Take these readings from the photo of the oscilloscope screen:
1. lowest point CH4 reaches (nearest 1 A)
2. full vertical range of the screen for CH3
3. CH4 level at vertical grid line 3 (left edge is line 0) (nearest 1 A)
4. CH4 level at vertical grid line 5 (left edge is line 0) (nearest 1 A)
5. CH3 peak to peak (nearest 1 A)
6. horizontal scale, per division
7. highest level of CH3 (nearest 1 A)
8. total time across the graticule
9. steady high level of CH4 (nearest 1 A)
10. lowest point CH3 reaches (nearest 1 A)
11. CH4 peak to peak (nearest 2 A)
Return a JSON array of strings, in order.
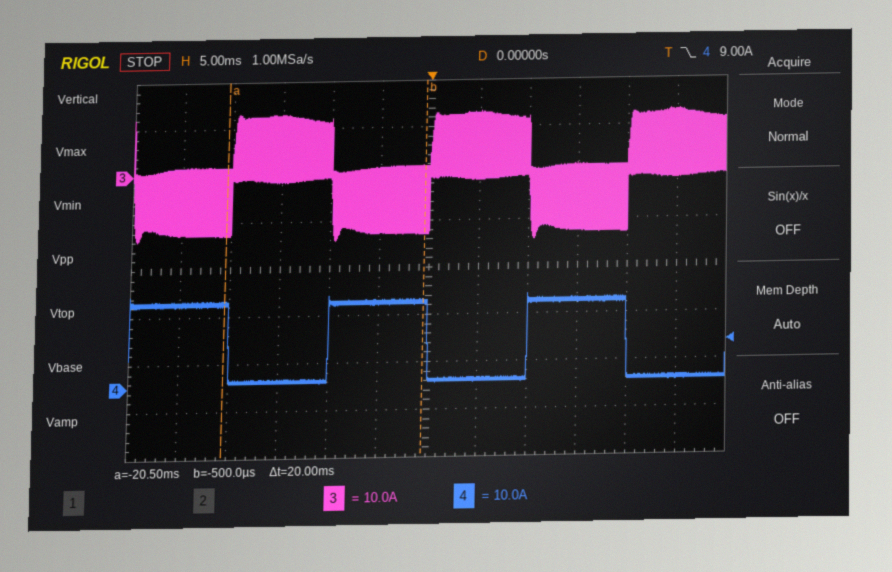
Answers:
["1 A", "80 A", "1 A", "18 A", "27 A", "5 ms", "13 A", "60 ms", "18 A", "-14 A", "18 A"]
